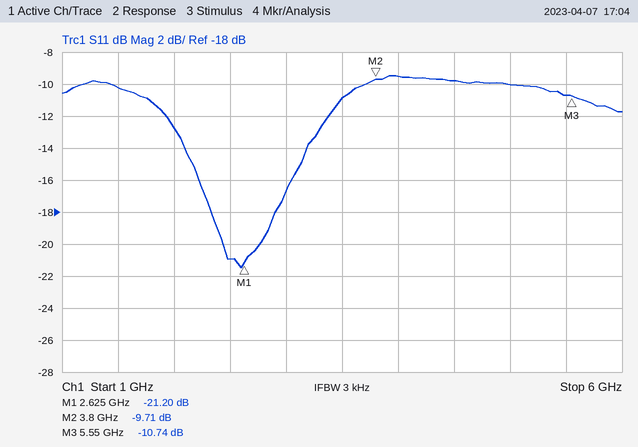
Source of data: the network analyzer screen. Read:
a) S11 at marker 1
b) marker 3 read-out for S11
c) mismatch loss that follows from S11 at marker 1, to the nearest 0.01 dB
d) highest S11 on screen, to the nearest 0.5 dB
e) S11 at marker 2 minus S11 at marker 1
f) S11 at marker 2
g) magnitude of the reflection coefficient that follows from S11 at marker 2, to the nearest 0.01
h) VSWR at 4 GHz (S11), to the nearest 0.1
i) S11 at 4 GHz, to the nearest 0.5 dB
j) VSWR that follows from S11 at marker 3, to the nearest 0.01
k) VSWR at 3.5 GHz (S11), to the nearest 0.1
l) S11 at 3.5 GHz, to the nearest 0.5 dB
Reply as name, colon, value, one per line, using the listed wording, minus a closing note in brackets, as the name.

S11 at marker 1: -21.20 dB
marker 3 read-out for S11: -10.74 dB
mismatch loss that follows from S11 at marker 1, to the nearest 0.01 dB: 0.03 dB
highest S11 on screen, to the nearest 0.5 dB: -9.5 dB
S11 at marker 2 minus S11 at marker 1: 11.49 dB
S11 at marker 2: -9.71 dB
magnitude of the reflection coefficient that follows from S11 at marker 2, to the nearest 0.01: 0.33
VSWR at 4 GHz (S11), to the nearest 0.1: 2.0
S11 at 4 GHz, to the nearest 0.5 dB: -9.5 dB
VSWR that follows from S11 at marker 3, to the nearest 0.01: 1.82
VSWR at 3.5 GHz (S11), to the nearest 0.1: 1.8
S11 at 3.5 GHz, to the nearest 0.5 dB: -11.0 dB
